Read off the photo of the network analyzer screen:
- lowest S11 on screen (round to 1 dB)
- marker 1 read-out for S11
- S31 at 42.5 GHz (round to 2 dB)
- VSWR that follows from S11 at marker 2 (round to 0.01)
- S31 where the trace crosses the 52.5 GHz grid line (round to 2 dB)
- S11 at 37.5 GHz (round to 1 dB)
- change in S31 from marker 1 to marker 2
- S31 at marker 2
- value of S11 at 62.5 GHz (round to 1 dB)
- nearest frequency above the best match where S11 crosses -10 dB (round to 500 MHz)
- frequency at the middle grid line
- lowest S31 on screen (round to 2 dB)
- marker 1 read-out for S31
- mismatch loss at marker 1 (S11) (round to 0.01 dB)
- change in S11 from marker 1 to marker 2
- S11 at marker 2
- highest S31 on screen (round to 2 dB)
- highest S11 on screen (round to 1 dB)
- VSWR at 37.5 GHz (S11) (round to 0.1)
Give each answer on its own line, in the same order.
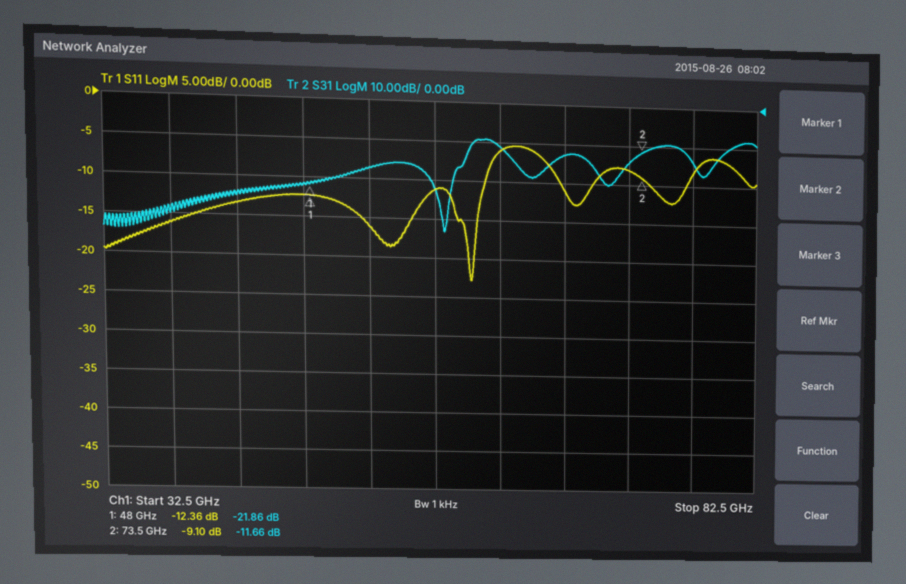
-23 dB
-12.36 dB
-24 dB
2.08
-18 dB
-16 dB
10.20 dB
-11.66 dB
-6 dB
61.5 GHz
57.5 GHz
-34 dB
-21.86 dB
0.26 dB
3.26 dB
-9.10 dB
-8 dB
-5 dB
1.4
